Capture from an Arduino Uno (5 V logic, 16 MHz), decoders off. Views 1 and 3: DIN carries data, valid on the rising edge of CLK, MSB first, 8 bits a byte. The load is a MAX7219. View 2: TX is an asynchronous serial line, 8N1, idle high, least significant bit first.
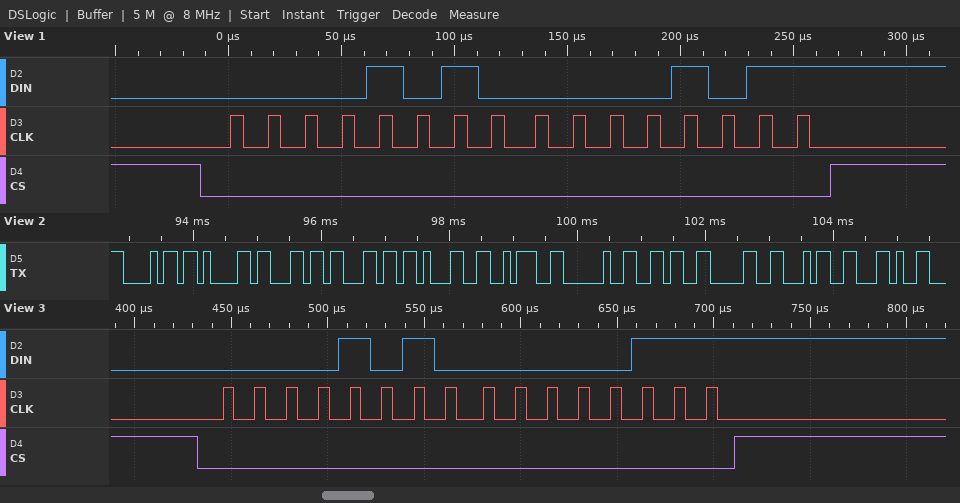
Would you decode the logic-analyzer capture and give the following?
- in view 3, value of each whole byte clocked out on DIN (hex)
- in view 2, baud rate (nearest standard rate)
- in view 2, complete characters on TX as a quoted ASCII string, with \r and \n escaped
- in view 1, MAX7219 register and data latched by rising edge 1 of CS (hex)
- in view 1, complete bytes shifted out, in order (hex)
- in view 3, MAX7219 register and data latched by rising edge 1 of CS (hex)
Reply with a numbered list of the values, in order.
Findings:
1. 0x0A 0x07
2. 9600 baud
3. "hall1: 604,"
4. register 0xA, data 0x0B
5. 0A 0B
6. register 0xA, data 0x07
